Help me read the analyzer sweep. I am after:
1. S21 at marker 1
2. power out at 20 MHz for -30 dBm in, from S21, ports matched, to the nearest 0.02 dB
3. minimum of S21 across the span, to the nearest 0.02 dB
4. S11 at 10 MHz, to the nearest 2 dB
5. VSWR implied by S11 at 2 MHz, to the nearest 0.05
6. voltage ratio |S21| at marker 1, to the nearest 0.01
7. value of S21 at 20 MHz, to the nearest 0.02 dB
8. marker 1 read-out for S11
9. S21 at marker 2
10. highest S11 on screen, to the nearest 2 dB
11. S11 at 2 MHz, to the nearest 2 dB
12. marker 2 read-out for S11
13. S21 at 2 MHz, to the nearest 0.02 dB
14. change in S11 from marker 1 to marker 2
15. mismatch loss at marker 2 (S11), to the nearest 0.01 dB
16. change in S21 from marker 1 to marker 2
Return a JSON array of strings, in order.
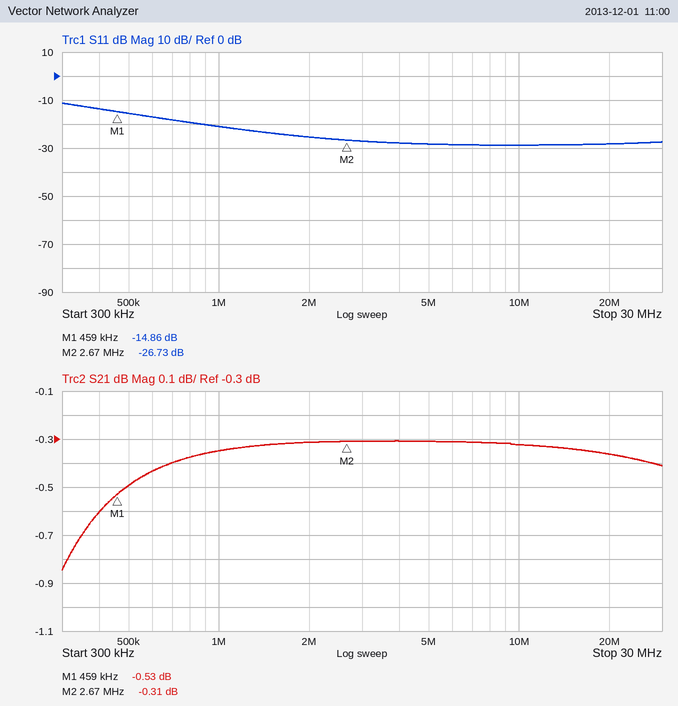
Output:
["-0.53 dB", "-30.36 dBm", "-0.84 dB", "-28 dB", "1.10", "0.94", "-0.36 dB", "-14.86 dB", "-0.31 dB", "-12 dB", "-26 dB", "-26.73 dB", "-0.32 dB", "-11.87 dB", "0.01 dB", "0.22 dB"]
